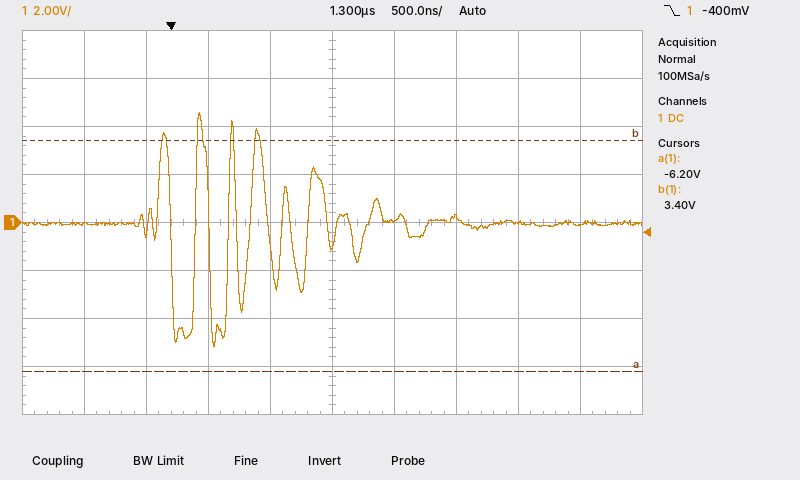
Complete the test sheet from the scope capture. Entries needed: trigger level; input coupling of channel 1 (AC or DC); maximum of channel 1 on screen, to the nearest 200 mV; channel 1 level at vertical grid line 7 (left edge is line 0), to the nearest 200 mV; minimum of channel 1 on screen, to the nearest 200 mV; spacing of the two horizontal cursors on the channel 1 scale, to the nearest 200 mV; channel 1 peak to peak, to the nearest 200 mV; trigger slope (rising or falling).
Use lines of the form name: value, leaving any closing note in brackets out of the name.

trigger level: -400 mV
input coupling of channel 1: DC
maximum of channel 1 on screen, to the nearest 200 mV: 4.6 V
channel 1 level at vertical grid line 7 (left edge is line 0), to the nearest 200 mV: 200 mV
minimum of channel 1 on screen, to the nearest 200 mV: -5.2 V
spacing of the two horizontal cursors on the channel 1 scale, to the nearest 200 mV: 9.6 V
channel 1 peak to peak, to the nearest 200 mV: 9.8 V
trigger slope: falling
